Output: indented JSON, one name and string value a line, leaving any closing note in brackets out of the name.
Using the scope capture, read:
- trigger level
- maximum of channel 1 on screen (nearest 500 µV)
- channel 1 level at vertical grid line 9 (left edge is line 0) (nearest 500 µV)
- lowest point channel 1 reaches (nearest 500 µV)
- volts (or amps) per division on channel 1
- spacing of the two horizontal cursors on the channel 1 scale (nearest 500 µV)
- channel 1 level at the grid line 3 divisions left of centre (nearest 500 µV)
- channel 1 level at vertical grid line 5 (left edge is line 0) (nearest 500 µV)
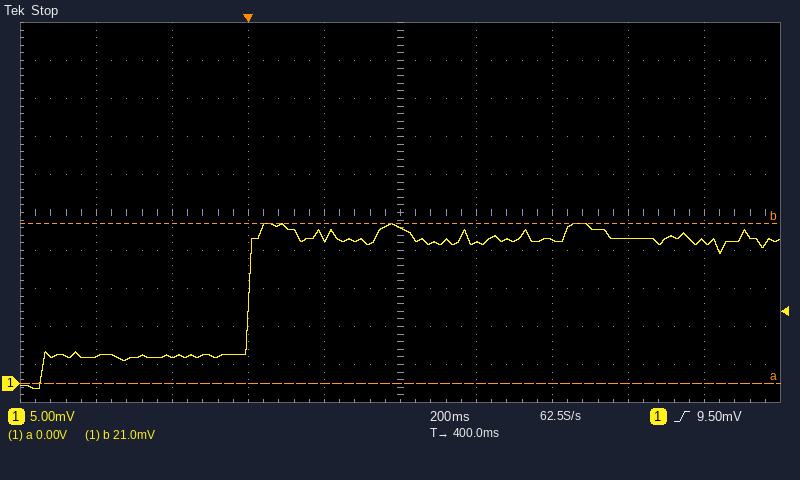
{
  "trigger level": "9.50 mV",
  "maximum of channel 1 on screen": "21.0 mV",
  "channel 1 level at vertical grid line 9 (left edge is line 0)": "18.5 mV",
  "lowest point channel 1 reaches": "-500 µV",
  "volts (or amps) per division on channel 1": "5 mV",
  "spacing of the two horizontal cursors on the channel 1 scale": "21.0 mV",
  "channel 1 level at the grid line 3 divisions left of centre": "3.5 mV",
  "channel 1 level at vertical grid line 5 (left edge is line 0)": "20.5 mV"
}
